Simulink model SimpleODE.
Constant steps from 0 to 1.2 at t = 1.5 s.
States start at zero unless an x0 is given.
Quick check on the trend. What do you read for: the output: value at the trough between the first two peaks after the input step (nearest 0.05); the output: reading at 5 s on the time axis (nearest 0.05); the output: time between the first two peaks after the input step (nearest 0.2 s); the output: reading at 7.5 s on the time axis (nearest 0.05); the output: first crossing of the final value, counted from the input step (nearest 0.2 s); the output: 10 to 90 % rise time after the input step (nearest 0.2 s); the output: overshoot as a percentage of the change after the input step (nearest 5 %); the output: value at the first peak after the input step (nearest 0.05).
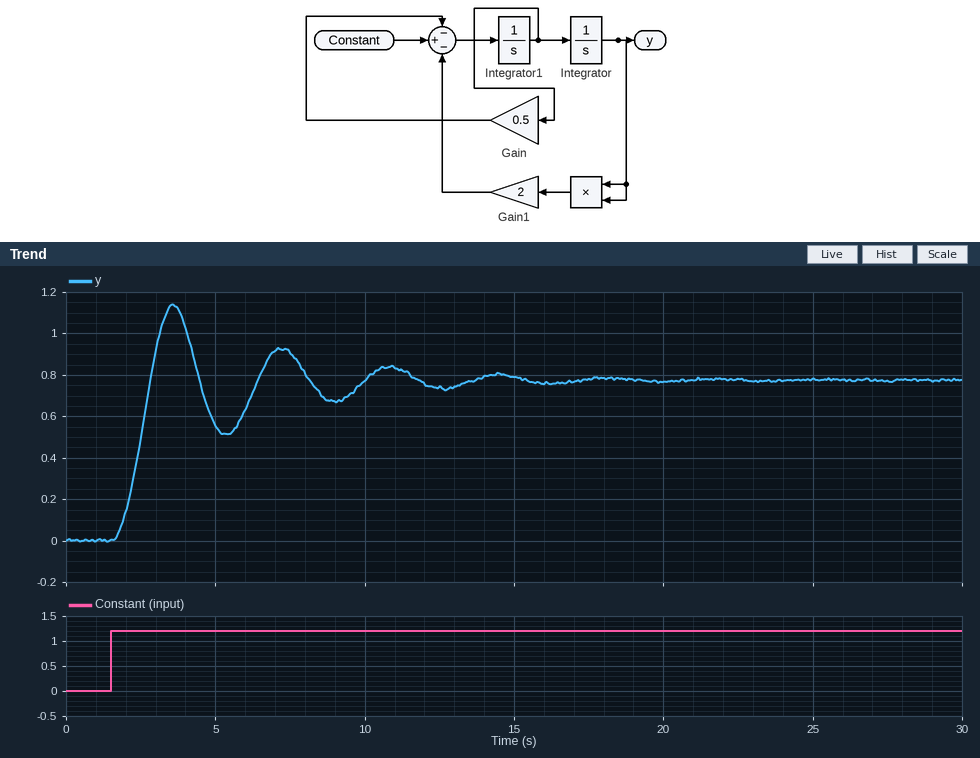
0.50
0.55
3.6 s
0.90
1.4 s
0.8 s
45 %
1.15
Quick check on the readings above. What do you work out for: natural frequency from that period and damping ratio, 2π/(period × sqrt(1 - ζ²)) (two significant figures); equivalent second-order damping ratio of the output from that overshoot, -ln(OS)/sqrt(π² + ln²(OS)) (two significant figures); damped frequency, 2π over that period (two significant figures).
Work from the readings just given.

1.8 rad/s
0.25
1.7 rad/s
